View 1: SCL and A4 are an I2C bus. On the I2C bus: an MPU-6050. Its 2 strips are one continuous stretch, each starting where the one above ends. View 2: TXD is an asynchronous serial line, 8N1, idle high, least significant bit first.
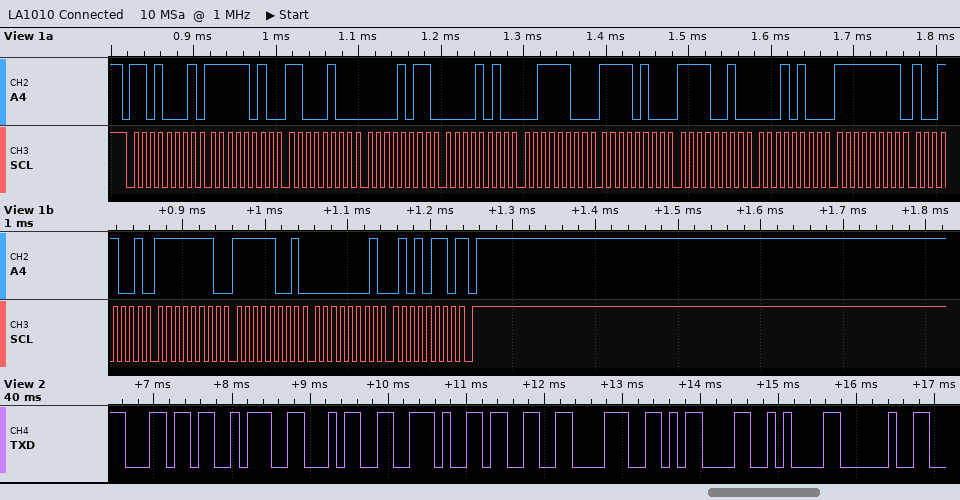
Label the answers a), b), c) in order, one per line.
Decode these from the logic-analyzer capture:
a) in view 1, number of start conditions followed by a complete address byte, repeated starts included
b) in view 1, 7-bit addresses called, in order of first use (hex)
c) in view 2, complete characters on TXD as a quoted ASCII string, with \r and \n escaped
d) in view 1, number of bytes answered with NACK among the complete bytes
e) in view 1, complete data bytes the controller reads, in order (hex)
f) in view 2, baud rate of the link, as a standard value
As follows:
a) 1
b) 0x68
c) "l:4.38\r\n "
d) 1
e) FA C4 0B 0A 3C F4 F2 14 FF 99 FE F9 01 56
f) 9600 baud
